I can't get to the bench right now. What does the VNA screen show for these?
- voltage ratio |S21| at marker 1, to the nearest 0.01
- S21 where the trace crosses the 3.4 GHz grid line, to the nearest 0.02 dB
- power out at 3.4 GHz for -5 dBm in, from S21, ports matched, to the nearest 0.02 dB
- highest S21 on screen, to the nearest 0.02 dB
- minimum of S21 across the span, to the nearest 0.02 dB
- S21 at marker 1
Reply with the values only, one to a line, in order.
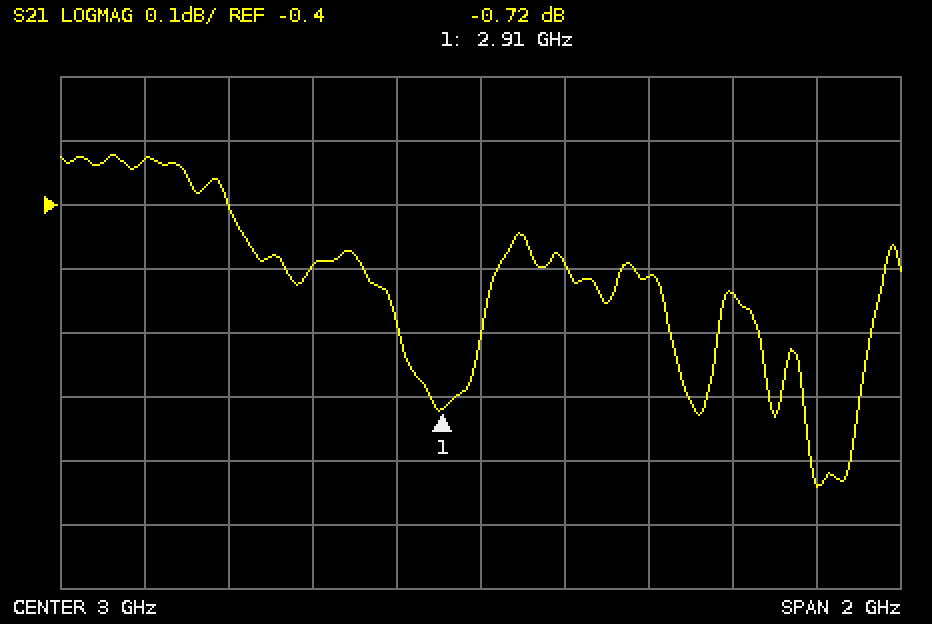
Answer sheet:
0.92
-0.52 dB
-5.52 dBm
-0.32 dB
-0.84 dB
-0.72 dB
